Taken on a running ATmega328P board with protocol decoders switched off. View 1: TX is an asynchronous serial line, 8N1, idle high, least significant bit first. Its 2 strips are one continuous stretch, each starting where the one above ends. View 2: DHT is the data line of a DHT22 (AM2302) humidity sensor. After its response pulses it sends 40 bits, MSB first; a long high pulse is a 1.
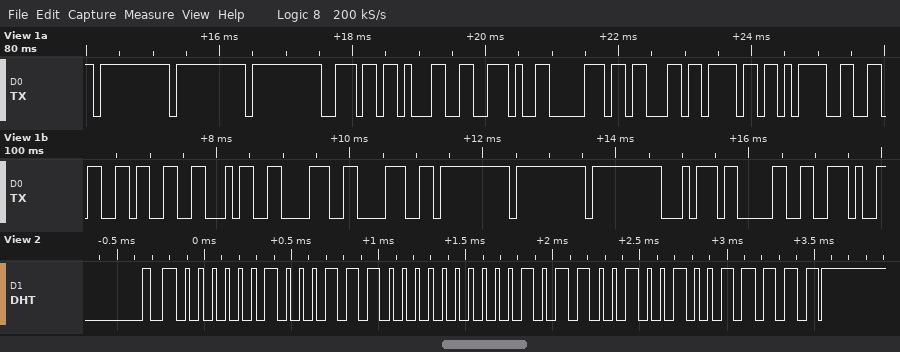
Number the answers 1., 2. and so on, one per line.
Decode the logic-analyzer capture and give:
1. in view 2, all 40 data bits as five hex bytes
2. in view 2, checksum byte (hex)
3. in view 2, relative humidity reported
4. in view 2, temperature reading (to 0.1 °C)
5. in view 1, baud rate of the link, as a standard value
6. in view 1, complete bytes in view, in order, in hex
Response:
1. 02 38 01 64 9F
2. 0x9F
3. 56.8 %
4. 35.6 °C
5. 9600 baud
6. FF FF FF 6E 31 2E 70 63 6F 3D 36 33 34 38 38 FF FF FF 74 30 2E
